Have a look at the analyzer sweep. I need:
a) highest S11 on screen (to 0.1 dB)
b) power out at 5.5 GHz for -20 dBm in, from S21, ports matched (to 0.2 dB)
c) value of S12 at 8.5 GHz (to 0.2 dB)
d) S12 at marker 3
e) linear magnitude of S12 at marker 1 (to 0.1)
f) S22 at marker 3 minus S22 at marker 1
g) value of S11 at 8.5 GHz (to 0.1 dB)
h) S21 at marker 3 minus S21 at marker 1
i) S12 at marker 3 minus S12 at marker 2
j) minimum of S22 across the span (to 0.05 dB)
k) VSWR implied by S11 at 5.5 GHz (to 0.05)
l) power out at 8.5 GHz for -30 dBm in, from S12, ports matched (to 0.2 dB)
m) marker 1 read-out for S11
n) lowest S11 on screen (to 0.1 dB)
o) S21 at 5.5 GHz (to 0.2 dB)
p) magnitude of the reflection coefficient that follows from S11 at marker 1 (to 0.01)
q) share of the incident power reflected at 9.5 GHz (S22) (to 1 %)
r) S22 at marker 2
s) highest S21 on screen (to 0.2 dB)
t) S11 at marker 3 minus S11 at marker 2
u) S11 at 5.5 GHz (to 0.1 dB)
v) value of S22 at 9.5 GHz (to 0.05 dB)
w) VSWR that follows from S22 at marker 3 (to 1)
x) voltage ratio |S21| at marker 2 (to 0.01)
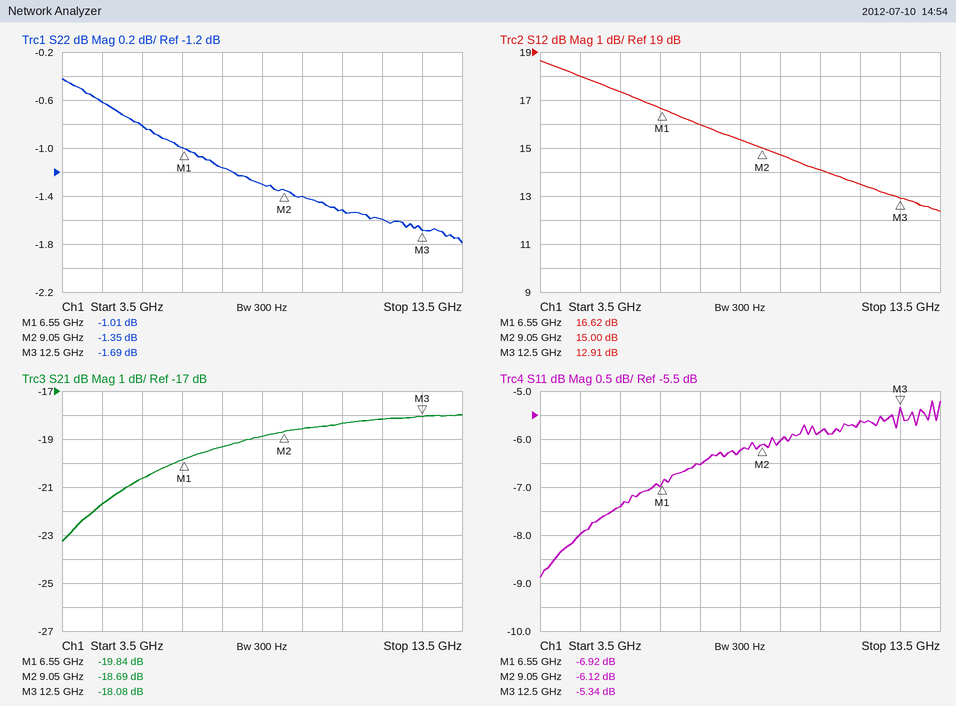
-5.2 dB
-40.6 dBm
15.4 dB
12.91 dB
6.8
-0.68 dB
-6.2 dB
1.76 dB
-2.09 dB
-1.80 dB
2.50
-14.6 dBm
-6.92 dB
-8.9 dB
-20.6 dB
0.45
72 %
-1.35 dB
-18.0 dB
0.78 dB
-7.4 dB
-1.40 dB
10
0.12
